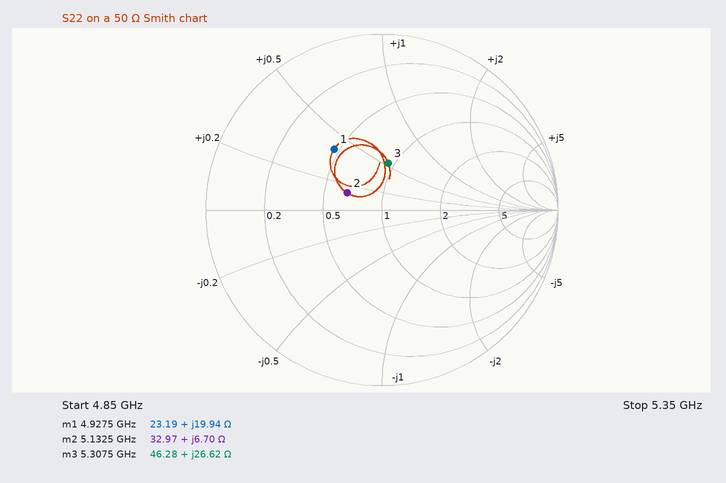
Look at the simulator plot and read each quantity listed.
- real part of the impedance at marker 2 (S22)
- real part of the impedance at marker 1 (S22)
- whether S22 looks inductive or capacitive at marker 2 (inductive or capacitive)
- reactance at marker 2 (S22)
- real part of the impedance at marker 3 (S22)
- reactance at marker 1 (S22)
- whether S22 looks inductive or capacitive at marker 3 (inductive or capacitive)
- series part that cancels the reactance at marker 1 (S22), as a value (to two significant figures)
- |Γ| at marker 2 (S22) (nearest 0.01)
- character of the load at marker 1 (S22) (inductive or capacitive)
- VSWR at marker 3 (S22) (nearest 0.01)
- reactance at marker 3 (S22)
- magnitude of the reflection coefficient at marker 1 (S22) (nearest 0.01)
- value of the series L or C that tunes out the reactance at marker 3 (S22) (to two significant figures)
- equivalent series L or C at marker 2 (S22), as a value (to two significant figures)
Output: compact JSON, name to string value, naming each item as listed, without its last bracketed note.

{"real part of the impedance at marker 2": "32.97 Ω", "real part of the impedance at marker 1": "23.19 Ω", "whether S22 looks inductive or capacitive at marker 2": "inductive", "reactance at marker 2": "+6.70 Ω", "real part of the impedance at marker 3": "46.28 Ω", "reactance at marker 1": "+19.94 Ω", "whether S22 looks inductive or capacitive at marker 3": "inductive", "series part that cancels the reactance at marker 1 (S22), as a value": "1.6 pF", "|Γ| at marker 2 (S22)": "0.22", "character of the load at marker 1 (S22)": "inductive", "VSWR at marker 3 (S22)": "1.74", "reactance at marker 3": "+26.62 Ω", "magnitude of the reflection coefficient at marker 1 (S22)": "0.44", "value of the series L or C that tunes out the reactance at marker 3 (S22)": "1.1 pF", "equivalent series L or C at marker 2 (S22), as a value": "210 pH"}
